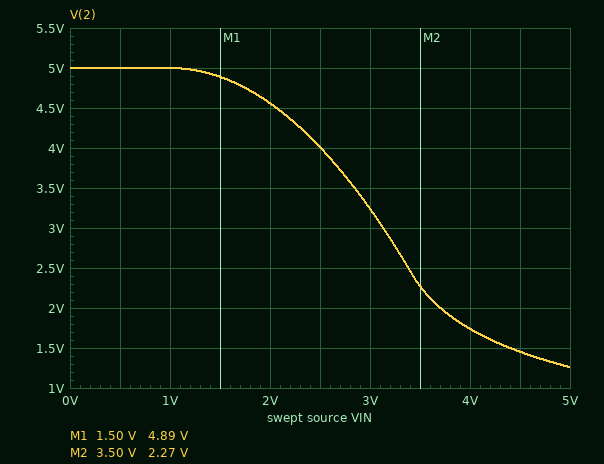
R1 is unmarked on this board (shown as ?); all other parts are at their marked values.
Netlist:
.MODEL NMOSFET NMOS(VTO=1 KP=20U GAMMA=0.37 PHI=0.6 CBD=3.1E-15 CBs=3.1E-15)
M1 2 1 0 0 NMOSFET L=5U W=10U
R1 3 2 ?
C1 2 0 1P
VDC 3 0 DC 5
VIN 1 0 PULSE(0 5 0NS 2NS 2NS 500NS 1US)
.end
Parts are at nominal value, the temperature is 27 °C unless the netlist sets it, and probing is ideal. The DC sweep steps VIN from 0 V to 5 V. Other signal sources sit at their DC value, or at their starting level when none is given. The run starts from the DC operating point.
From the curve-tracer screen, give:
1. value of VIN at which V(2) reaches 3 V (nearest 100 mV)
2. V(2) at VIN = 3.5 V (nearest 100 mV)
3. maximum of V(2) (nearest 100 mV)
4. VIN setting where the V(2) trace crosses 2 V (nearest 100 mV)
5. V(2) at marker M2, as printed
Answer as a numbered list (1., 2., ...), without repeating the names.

1. 3.1 V
2. 2.3 V
3. 5.0 V
4. 3.7 V
5. 2.27 V
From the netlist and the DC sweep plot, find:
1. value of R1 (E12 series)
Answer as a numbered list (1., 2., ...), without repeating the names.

1. 22 kΩ
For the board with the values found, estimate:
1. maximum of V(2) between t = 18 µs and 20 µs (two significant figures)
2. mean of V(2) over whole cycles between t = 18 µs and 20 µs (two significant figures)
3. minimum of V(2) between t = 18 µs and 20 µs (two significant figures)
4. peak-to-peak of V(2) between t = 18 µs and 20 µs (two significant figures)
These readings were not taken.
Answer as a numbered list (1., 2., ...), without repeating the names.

1. 5.0 V
2. 3.1 V
3. 1.3 V
4. 3.7 V
